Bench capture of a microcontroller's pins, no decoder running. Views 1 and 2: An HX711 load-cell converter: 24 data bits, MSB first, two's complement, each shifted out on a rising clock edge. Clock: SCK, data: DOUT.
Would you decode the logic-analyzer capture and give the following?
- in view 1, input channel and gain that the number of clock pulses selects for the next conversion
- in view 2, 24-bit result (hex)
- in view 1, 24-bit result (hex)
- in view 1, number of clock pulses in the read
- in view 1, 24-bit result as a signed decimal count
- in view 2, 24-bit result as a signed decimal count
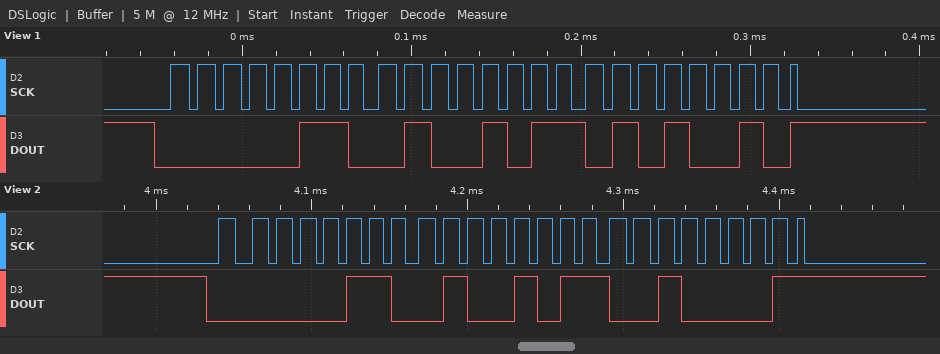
channel A, gain 128
0x064B21
0x064B52
25
412498
412449
